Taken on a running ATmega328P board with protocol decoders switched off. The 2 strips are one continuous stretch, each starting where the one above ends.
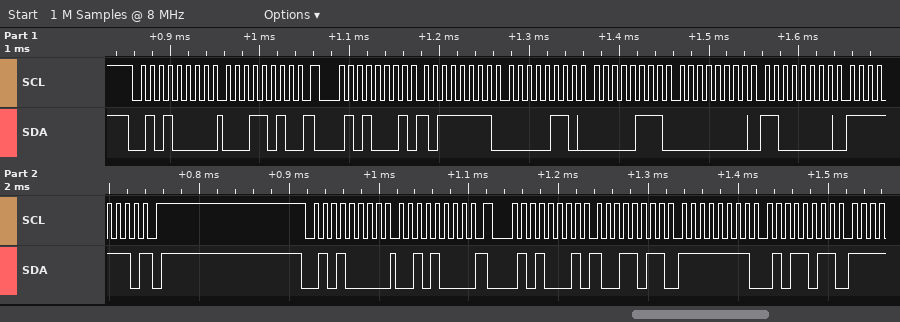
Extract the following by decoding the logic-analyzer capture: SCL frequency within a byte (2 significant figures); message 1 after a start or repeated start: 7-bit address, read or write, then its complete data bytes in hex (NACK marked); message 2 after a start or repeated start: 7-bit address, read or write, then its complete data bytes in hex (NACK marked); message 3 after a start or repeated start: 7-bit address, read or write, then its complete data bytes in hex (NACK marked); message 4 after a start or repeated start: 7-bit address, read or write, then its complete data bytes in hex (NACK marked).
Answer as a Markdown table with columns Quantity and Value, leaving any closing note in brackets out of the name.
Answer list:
| Quantity | Value |
|---|---|
| SCL frequency within a byte | 100 kHz |
| message 1 after a start or repeated start: 7-bit address, read or write, then its complete data bytes in hex | 0x28 write: 1A |
| message 2 after a start or repeated start: 7-bit address, read or write, then its complete data bytes in hex | 0x28 read: BF 06 07 00 C0 FE NACK |
| message 3 after a start or repeated start: 7-bit address, read or write, then its complete data bytes in hex | 0x28 write: 28 |
| message 4 after a start or repeated start: 7-bit address, read or write, then its complete data bytes in hex | 0x28 read: 9B FF 5B |
